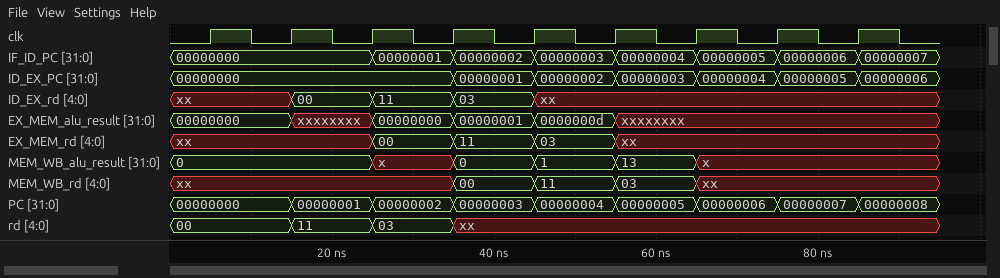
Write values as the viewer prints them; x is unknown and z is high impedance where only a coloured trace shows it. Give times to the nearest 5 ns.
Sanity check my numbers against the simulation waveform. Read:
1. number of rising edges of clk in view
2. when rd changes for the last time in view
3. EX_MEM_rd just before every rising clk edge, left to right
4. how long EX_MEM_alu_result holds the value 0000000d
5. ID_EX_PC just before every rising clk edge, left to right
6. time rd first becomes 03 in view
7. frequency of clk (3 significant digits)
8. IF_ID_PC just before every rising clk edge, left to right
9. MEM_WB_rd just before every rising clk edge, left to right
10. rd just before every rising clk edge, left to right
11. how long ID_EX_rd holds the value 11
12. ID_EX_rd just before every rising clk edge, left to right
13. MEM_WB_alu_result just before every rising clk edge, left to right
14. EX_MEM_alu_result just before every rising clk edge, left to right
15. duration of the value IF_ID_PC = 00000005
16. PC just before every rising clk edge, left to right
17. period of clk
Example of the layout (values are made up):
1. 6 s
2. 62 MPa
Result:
1. 9
2. 35 ns
3. xx, xx, xx, 00, 11, 03, xx, xx, xx
4. 10 ns
5. 00000000, 00000000, 00000000, 00000000, 00000001, 00000002, 00000003, 00000004, 00000005
6. 25 ns
7. 100 MHz
8. 00000000, 00000000, 00000000, 00000001, 00000002, 00000003, 00000004, 00000005, 00000006
9. xx, xx, xx, xx, 00, 11, 03, xx, xx
10. 00, 00, 11, 03, xx, xx, xx, xx, xx
11. 10 ns
12. xx, xx, 00, 11, 03, xx, xx, xx, xx
13. 0, 0, 0, x, 0, 1, 13, x, x
14. 00000000, 00000000, xxxxxxxx, 00000000, 00000001, 0000000d, xxxxxxxx, xxxxxxxx, xxxxxxxx
15. 10 ns
16. 00000000, 00000000, 00000001, 00000002, 00000003, 00000004, 00000005, 00000006, 00000007
17. 10 ns
